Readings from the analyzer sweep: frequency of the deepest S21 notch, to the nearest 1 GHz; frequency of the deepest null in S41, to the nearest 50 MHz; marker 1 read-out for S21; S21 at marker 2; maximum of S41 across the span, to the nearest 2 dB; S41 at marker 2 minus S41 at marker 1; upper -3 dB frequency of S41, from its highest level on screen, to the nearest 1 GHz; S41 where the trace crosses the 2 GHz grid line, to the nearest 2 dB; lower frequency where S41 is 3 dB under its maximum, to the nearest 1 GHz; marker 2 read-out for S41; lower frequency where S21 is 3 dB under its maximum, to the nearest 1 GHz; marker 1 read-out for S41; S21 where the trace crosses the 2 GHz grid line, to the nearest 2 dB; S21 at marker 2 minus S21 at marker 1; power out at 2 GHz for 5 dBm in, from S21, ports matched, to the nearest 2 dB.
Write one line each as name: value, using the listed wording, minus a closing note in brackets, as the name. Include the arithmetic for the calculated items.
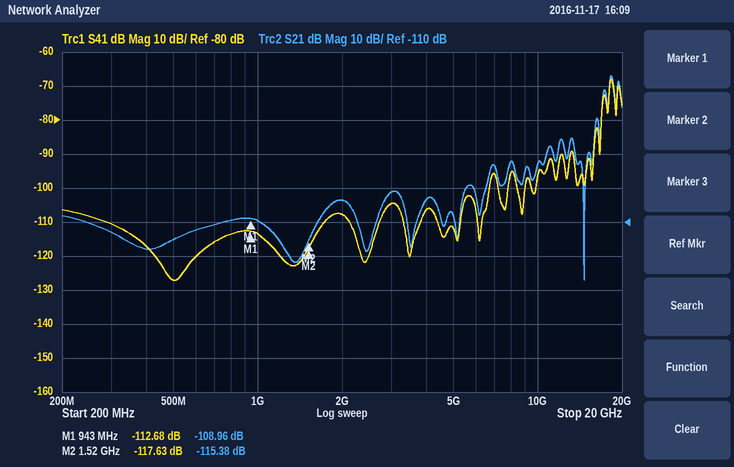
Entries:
frequency of the deepest S21 notch, to the nearest 1 GHz: 15 GHz
frequency of the deepest null in S41, to the nearest 50 MHz: 500 MHz
marker 1 read-out for S21: -108.96 dB
S21 at marker 2: -115.38 dB
maximum of S41 across the span, to the nearest 2 dB: -68 dB
S41 at marker 2 minus S41 at marker 1: -117.63 − (-112.68) = -4.95 dB
upper -3 dB frequency of S41, from its highest level on screen, to the nearest 1 GHz: 19 GHz
S41 where the trace crosses the 2 GHz grid line, to the nearest 2 dB: -108 dB
lower frequency where S41 is 3 dB under its maximum, to the nearest 1 GHz: 18 GHz
marker 2 read-out for S41: -117.63 dB
lower frequency where S21 is 3 dB under its maximum, to the nearest 1 GHz: 18 GHz
marker 1 read-out for S41: -112.68 dB
S21 where the trace crosses the 2 GHz grid line, to the nearest 2 dB: -104 dB
S21 at marker 2 minus S21 at marker 1: -115.38 − (-108.96) = -6.42 dB
power out at 2 GHz for 5 dBm in, from S21, ports matched, to the nearest 2 dB: 5 dBm + (-104 dB) = -98 dBm
